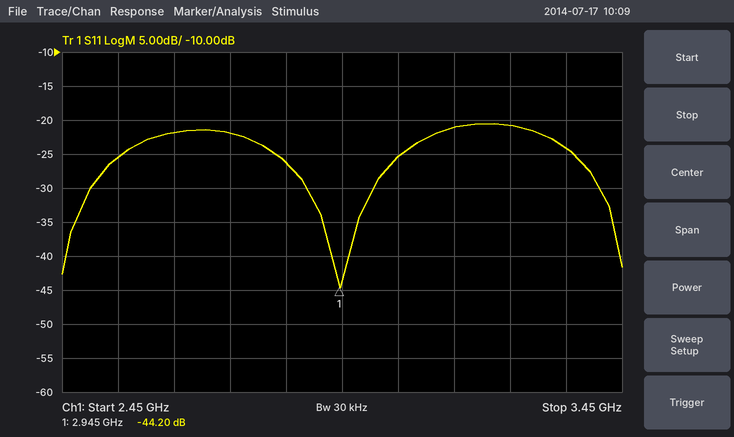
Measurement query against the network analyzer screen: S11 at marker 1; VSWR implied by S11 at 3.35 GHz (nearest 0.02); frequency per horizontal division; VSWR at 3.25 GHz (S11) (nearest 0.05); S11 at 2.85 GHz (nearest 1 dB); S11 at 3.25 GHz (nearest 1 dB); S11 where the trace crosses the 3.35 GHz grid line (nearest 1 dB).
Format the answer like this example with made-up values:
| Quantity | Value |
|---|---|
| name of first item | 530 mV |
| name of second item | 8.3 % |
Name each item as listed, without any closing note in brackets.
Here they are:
| Quantity | Value |
|---|---|
| S11 at marker 1 | -44.20 dB |
| VSWR implied by S11 at 3.35 GHz | 1.14 |
| frequency per horizontal division | 100 MHz |
| VSWR at 3.25 GHz (S11) | 1.20 |
| S11 at 2.85 GHz | -26 dB |
| S11 at 3.25 GHz | -21 dB |
| S11 where the trace crosses the 3.35 GHz grid line | -24 dB |
